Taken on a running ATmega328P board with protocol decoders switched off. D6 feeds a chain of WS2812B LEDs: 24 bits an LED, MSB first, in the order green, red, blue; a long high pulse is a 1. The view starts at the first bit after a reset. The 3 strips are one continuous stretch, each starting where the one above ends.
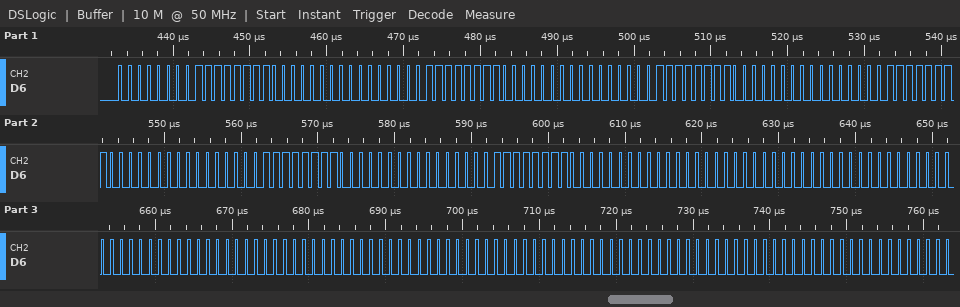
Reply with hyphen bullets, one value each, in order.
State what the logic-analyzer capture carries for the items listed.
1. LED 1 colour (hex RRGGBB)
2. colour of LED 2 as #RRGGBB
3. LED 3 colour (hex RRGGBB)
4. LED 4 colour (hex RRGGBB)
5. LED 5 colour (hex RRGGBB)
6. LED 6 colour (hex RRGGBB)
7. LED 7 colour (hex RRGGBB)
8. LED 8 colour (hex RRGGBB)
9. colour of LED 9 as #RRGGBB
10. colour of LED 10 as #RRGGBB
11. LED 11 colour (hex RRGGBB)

- #FF0000
- #FF0000
- #FF0000
- #FF0000
- #FF0000
- #FF0000
- #000000
- #000000
- #000000
- #000000
- #000000
